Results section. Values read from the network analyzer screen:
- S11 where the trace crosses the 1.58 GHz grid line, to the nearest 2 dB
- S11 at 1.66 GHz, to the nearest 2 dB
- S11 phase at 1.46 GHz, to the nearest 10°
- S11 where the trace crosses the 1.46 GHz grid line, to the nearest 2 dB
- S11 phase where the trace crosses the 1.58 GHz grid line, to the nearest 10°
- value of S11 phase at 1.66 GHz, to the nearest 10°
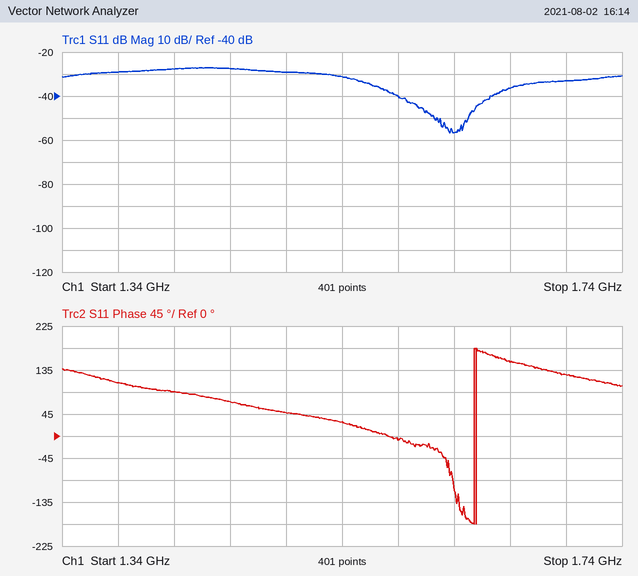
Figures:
-40 dB
-36 dB
70°
-28 dB
-10°
150°
